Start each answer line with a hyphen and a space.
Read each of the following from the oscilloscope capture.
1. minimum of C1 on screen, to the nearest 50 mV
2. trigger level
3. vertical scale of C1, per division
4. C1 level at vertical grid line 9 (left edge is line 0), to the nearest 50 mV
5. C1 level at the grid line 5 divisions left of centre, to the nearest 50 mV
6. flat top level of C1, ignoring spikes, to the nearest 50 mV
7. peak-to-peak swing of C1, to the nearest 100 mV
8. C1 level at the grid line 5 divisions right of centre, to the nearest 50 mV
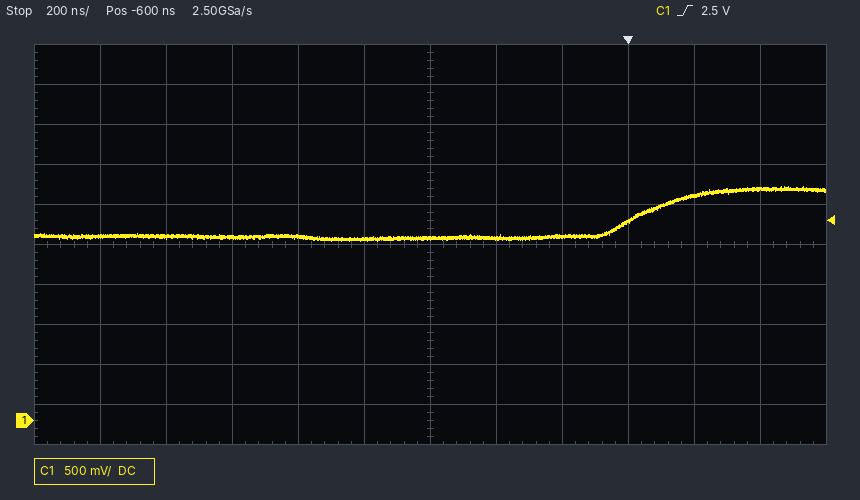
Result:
- 2.25 V
- 2.5 V
- 500 mV
- 2.50 V
- 2.30 V
- 2.90 V
- 700 mV
- 2.90 V
